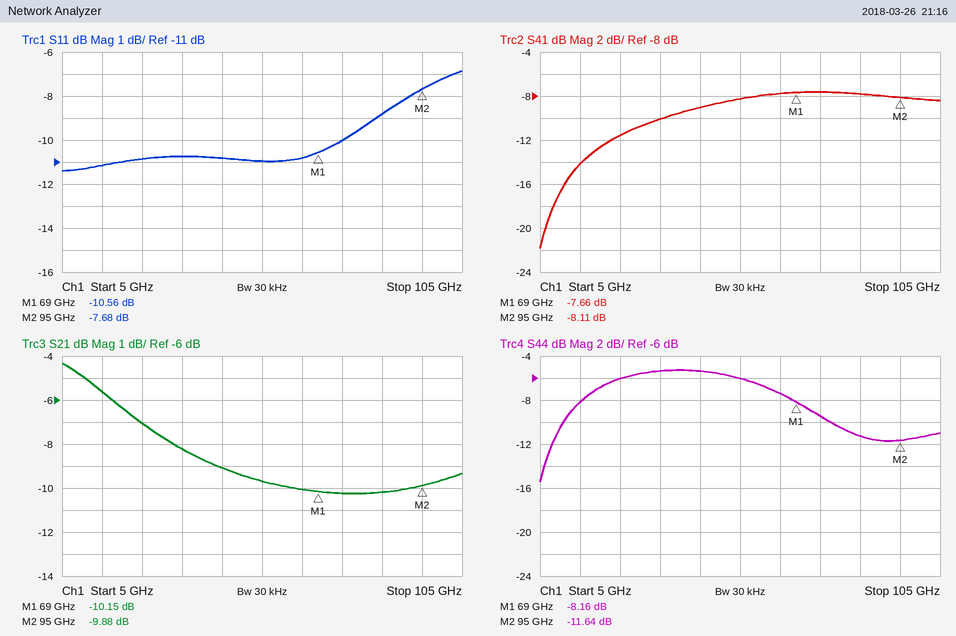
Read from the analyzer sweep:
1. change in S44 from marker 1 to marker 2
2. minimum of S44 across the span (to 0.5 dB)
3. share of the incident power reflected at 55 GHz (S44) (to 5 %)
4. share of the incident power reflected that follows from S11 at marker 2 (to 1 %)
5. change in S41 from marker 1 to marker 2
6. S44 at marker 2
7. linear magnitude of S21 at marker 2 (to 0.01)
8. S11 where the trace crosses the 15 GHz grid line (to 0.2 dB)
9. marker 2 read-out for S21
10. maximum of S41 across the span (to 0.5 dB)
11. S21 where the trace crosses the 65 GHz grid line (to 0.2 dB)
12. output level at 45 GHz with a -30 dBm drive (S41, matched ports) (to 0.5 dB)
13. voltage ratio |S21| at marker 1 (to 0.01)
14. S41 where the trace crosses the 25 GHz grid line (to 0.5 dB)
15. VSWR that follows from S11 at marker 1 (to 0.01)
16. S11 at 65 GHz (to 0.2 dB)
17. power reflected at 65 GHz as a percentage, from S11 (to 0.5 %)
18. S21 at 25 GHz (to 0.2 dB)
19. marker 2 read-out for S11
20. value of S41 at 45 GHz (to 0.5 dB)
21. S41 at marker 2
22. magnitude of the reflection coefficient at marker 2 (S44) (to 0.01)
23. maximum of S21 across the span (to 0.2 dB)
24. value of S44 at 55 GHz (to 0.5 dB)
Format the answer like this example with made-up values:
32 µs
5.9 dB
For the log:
-3.48 dB
-15.5 dB
25 %
17 %
-0.45 dB
-11.64 dB
0.32
-11.2 dB
-9.88 dB
-7.5 dB
-10.0 dB
-39.0 dBm
0.31
-11.5 dB
1.84
-10.8 dB
8.5 %
-7.0 dB
-7.68 dB
-9.0 dB
-8.11 dB
0.26
-4.4 dB
-6.0 dB
